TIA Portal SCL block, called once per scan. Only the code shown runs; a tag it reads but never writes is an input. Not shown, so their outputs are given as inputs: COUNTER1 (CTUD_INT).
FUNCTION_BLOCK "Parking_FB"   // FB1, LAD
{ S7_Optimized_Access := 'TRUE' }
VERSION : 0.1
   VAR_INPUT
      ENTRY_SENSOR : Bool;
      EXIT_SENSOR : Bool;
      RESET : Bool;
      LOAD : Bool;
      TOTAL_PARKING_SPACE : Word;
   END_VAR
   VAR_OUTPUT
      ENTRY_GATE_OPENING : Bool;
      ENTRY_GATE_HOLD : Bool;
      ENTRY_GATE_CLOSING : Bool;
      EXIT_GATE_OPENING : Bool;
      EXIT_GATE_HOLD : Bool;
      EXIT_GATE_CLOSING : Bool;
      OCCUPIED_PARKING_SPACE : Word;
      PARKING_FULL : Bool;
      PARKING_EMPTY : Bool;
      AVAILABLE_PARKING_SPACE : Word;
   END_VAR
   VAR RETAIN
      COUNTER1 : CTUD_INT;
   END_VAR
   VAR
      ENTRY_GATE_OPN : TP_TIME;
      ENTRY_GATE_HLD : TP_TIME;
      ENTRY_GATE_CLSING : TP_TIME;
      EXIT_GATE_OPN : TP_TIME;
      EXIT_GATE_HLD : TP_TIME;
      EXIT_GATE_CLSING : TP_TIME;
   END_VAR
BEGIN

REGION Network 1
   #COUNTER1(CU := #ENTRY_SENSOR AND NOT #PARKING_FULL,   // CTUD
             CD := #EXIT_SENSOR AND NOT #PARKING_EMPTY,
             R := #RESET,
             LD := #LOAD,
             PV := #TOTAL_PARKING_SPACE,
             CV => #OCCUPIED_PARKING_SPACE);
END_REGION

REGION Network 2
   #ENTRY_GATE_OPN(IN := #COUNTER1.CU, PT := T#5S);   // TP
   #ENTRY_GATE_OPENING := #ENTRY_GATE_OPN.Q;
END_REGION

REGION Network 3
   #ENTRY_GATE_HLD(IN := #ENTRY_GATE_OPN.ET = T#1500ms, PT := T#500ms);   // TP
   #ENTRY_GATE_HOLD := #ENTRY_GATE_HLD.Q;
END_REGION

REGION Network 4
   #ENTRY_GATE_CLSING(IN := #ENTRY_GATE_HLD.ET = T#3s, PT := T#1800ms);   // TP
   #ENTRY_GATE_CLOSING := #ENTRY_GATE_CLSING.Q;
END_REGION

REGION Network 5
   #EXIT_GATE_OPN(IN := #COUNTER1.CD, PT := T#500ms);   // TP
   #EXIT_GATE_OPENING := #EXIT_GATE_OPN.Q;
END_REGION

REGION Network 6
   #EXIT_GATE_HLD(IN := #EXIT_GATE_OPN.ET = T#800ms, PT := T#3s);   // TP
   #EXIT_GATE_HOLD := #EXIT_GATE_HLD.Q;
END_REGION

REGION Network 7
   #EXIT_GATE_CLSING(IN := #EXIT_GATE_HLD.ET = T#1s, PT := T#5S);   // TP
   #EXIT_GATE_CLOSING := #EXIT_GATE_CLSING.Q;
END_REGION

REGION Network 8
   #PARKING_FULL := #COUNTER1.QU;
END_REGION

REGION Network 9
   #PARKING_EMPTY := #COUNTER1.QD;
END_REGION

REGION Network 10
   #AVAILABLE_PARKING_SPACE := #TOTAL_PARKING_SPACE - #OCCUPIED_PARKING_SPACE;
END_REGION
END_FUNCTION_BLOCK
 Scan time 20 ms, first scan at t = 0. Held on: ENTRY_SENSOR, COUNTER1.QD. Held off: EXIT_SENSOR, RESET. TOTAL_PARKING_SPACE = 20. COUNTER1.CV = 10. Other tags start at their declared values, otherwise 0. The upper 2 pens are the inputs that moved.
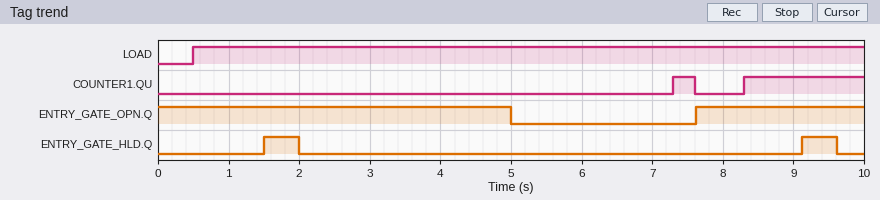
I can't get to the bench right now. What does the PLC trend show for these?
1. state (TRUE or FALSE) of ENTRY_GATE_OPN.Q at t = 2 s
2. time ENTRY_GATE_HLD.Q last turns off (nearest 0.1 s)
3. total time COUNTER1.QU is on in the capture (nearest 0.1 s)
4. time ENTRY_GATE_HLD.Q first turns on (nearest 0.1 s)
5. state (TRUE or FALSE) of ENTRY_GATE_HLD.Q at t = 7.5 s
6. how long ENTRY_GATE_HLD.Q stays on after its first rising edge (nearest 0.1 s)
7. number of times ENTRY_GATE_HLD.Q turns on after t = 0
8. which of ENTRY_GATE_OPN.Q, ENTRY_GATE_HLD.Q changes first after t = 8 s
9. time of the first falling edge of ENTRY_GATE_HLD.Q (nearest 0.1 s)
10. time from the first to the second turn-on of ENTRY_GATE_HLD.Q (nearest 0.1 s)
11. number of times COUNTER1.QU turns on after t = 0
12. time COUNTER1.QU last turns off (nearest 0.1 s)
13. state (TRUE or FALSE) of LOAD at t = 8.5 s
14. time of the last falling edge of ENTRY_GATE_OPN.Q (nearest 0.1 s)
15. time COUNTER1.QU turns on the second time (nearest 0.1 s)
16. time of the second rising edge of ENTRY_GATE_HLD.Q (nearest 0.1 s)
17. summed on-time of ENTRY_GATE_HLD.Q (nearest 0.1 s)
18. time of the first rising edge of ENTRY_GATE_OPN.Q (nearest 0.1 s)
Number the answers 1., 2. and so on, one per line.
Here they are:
1. TRUE
2. 9.6 s
3. 2.0 s
4. 1.5 s
5. FALSE
6. 0.5 s
7. 2
8. ENTRY_GATE_HLD.Q
9. 2.0 s
10. 7.6 s
11. 2
12. 7.6 s
13. TRUE
14. 5.0 s
15. 8.3 s
16. 9.1 s
17. 1.0 s
18. 7.6 s
